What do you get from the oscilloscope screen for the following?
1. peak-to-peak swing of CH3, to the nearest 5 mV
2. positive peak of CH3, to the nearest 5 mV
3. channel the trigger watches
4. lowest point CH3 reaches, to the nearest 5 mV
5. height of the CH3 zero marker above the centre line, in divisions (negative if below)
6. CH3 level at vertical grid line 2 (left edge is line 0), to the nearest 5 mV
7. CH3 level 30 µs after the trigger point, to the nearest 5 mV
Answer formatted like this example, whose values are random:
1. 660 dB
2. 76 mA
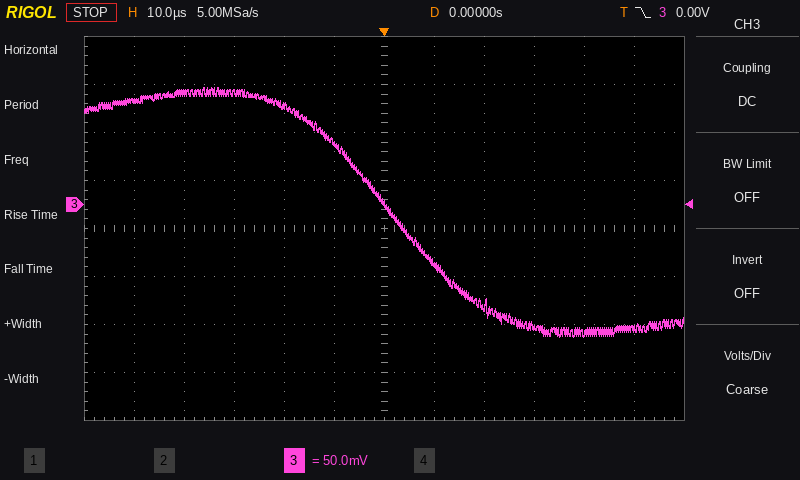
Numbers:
1. 260 mV
2. 120 mV
3. CH3
4. -140 mV
5. +0.5 div
6. 115 mV
7. -125 mV
